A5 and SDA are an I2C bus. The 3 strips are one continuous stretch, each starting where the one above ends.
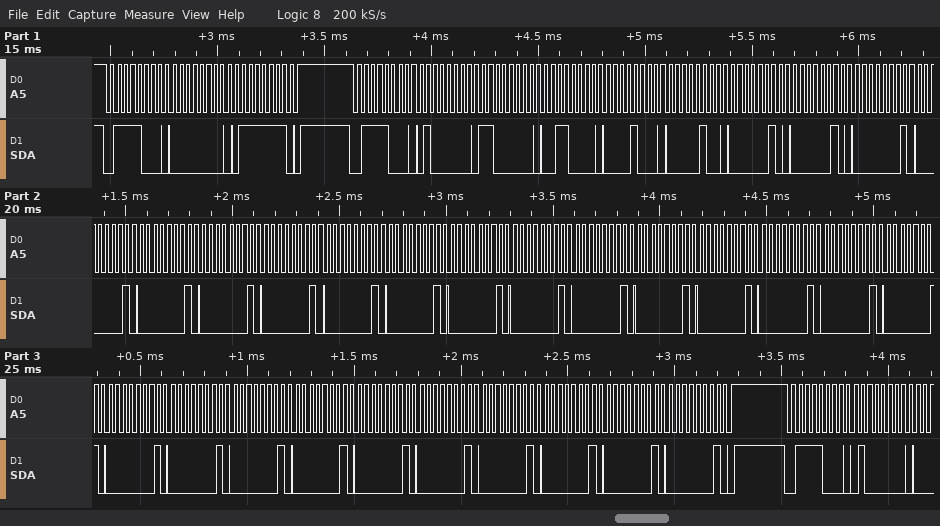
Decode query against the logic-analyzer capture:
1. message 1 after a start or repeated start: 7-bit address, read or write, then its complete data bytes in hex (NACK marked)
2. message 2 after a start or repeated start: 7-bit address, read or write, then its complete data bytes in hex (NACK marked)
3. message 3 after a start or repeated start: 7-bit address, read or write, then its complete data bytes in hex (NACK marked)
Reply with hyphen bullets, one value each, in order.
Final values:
- 0x3C write: 00 7F
- 0x3C write: 40 C0 30 08 04 02 02 01 01 01 01 01 01 01 01 01 01 01 01 01 01 01 01 01 01 01 01 01 01 01 01 01
- 0x3C write: 40
